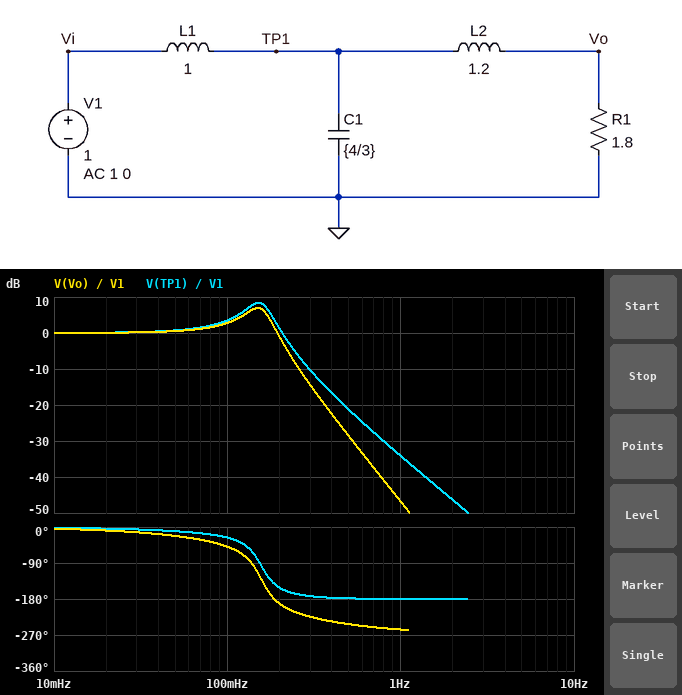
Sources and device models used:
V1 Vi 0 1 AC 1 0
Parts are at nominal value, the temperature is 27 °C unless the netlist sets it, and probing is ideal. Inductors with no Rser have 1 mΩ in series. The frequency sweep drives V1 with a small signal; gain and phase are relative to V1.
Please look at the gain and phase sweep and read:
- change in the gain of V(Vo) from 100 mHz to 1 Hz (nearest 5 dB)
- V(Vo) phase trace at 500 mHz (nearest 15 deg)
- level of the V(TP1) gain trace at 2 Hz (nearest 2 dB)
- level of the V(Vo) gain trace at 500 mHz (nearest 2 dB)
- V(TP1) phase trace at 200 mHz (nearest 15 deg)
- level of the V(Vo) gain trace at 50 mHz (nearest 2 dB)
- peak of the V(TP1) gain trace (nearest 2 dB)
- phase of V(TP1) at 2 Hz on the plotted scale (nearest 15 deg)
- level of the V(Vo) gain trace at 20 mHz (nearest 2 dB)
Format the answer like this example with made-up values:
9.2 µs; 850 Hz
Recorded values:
-50 dB; -240 deg; -46 dB; -28 dB; -150 deg; 0 dB; 8 dB; -180 deg; 0 dB
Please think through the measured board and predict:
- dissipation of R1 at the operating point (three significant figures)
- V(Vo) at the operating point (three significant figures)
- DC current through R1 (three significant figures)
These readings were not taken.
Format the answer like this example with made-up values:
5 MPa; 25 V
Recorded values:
554 mW; 999 mV; 555 mA
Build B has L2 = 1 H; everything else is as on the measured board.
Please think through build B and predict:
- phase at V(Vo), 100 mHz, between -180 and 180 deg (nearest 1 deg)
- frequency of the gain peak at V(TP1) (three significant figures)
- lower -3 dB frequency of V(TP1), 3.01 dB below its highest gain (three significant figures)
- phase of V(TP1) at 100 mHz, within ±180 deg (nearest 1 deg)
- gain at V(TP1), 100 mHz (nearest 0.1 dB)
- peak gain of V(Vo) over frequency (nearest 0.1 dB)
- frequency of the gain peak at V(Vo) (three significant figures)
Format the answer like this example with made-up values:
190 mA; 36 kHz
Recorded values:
-47 deg; 149 mHz; 112 mHz; -28 deg; 3.6 dB; 6.7 dB; 147 mHz
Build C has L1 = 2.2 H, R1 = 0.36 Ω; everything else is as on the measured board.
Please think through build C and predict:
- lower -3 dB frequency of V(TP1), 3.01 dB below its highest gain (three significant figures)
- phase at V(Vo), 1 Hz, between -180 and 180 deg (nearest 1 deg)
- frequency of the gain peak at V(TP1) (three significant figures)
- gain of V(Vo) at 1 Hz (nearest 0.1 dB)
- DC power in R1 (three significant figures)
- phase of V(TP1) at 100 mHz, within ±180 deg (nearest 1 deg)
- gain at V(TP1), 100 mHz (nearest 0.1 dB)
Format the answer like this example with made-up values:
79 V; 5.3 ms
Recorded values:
137 mHz; 93 deg; 153 mHz; -67.5 dB; 2.75 W; -28 deg; -3.6 dB
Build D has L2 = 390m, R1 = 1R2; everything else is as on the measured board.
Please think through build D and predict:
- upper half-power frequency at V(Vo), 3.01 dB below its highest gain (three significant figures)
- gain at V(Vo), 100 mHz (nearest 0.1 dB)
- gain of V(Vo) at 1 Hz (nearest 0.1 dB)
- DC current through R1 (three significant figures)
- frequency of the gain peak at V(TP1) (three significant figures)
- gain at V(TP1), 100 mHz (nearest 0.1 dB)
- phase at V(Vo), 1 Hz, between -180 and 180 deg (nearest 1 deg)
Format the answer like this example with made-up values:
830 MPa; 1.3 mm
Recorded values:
183 mHz; 2.1 dB; -41.0 dB; 832 mA; 134 mHz; 2.3 dB; 117 deg
